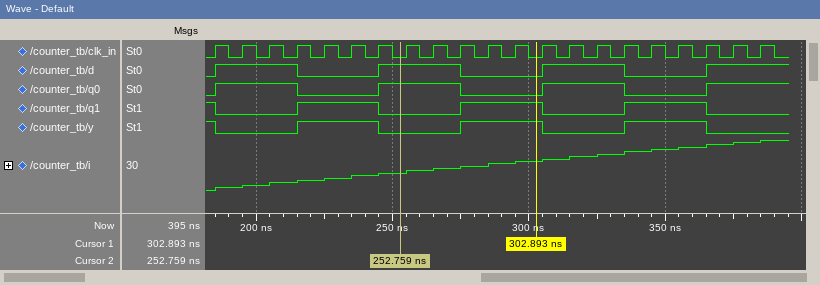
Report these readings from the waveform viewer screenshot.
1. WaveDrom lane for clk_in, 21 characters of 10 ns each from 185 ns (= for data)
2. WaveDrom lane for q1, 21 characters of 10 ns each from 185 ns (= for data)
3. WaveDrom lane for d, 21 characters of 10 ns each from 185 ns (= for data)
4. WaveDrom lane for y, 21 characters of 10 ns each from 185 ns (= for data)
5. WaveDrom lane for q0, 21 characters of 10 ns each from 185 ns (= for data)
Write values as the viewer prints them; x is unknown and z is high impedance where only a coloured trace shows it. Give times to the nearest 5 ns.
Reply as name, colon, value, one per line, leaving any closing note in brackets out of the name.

WaveDrom lane for clk_in, 21 characters of 10 ns each from 185 ns: {name: 'clk_in', wave: 'p....................'}
WaveDrom lane for q1, 21 characters of 10 ns each from 185 ns: {name: 'q1', wave: '0..1..0..1..0..1..0..'}
WaveDrom lane for d, 21 characters of 10 ns each from 185 ns: {name: 'd', wave: '1..0..1..0..1..0..1..'}
WaveDrom lane for y, 21 characters of 10 ns each from 185 ns: {name: 'y', wave: '0..1..0..1..0..1..0..'}
WaveDrom lane for q0, 21 characters of 10 ns each from 185 ns: {name: 'q0', wave: '1..0..1..0..1..0..1..'}
